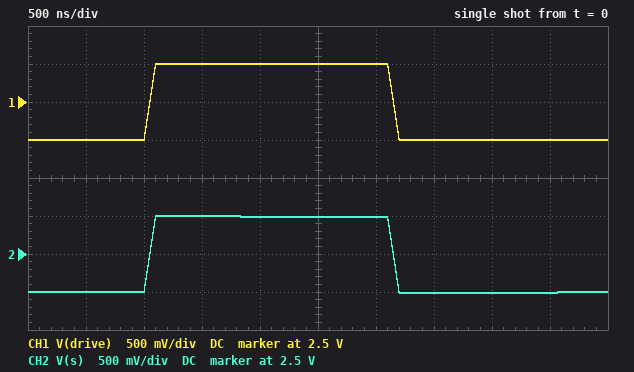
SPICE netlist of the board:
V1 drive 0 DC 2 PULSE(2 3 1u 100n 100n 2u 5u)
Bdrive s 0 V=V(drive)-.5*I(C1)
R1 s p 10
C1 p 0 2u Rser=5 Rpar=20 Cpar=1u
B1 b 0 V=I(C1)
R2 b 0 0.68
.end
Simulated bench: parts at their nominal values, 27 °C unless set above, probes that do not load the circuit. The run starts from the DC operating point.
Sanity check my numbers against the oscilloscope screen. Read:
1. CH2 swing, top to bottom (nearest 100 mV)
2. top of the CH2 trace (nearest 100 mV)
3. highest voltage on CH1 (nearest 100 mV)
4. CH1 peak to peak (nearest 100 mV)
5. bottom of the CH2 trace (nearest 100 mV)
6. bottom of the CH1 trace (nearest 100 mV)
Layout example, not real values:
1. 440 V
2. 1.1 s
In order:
1. 1.0 V
2. 3.0 V
3. 3.0 V
4. 1.0 V
5. 2.0 V
6. 2.0 V
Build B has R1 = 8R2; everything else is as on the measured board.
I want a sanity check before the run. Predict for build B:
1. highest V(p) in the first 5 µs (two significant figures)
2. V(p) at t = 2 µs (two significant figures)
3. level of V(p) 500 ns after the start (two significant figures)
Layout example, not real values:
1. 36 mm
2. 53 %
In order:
1. 1.6 V
2. 1.5 V
3. 1.4 V
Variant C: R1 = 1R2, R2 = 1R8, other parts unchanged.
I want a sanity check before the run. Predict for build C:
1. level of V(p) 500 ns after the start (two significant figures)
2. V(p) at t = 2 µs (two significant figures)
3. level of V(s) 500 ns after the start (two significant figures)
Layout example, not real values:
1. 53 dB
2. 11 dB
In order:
1. 1.9 V
2. 2.4 V
3. 2.0 V
